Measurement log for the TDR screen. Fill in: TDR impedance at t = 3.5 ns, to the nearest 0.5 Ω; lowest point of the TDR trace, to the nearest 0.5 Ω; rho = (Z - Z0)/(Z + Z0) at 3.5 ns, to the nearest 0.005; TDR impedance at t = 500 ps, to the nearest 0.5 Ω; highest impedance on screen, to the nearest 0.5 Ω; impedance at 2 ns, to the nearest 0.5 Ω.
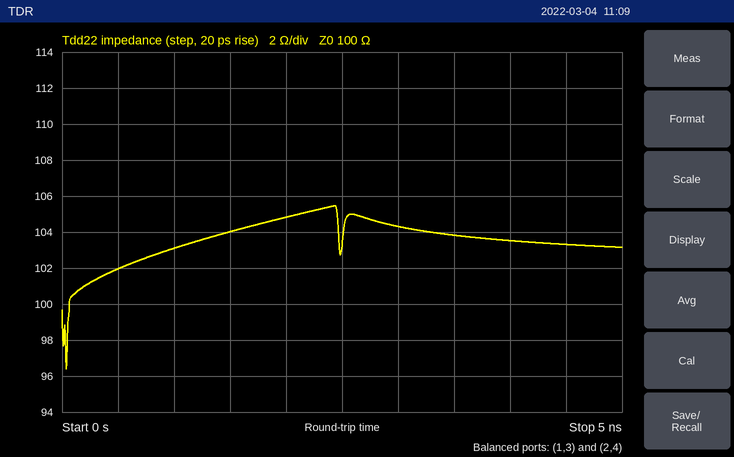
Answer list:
104.0 Ω
96.5 Ω
+0.020
102.0 Ω
105.5 Ω
105.0 Ω
